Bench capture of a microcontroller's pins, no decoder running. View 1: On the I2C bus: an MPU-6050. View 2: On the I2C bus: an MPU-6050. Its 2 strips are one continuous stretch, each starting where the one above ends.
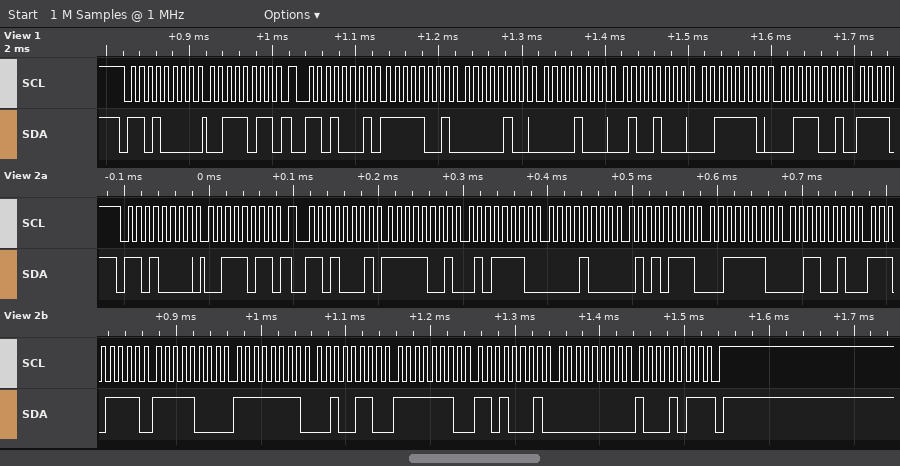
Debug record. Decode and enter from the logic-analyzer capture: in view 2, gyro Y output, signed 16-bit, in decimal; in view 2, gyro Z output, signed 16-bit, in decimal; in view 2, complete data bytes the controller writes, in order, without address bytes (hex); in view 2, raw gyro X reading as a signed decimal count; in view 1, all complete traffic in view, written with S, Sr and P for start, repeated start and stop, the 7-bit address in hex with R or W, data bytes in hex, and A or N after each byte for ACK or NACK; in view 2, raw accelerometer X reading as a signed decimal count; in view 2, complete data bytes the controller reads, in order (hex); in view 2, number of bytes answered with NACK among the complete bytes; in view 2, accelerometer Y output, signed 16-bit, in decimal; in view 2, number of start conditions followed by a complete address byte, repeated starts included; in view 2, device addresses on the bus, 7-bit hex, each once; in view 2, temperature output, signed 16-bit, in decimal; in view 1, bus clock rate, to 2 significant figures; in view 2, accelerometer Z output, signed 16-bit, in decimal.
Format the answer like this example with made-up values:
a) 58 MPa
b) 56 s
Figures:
a) -303
b) 139
c) 3B
d) -218
e) S 68W A 3B A Sr 68R A F9 A 04 A 08 A 48 A 3E A 39 A
f) -1698
g) F9 5E 08 57 3E 32 EF F8 FF 26 FE D1 00 8B
h) 1
i) 2135
j) 2
k) 0x68
l) -4104
m) 100 kHz
n) 15922
